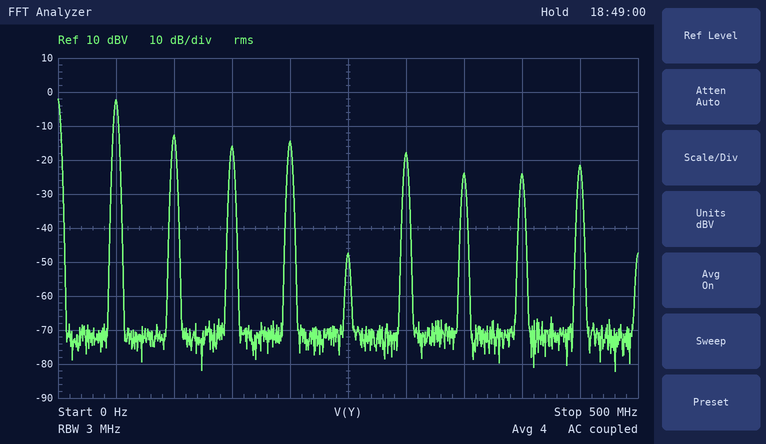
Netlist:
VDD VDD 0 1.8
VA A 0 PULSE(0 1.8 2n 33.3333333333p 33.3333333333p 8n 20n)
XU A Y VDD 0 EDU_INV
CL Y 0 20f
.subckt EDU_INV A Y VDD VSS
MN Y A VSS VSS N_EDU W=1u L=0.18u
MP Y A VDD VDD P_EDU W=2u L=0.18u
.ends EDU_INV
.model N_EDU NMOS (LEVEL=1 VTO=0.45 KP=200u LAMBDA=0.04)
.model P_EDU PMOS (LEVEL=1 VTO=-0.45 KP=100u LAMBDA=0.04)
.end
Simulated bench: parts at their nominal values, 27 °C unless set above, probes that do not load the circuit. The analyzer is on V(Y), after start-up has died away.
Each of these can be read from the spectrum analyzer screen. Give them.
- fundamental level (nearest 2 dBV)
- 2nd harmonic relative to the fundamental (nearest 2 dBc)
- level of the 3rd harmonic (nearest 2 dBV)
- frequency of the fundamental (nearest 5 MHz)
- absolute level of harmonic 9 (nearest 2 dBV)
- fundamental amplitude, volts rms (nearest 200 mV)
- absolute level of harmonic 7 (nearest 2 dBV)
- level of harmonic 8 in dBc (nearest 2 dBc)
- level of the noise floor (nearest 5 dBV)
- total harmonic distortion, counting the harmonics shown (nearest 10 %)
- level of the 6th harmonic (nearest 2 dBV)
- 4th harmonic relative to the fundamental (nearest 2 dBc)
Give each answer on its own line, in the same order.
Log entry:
-2 dBV
-10 dBc
-16 dBV
50 MHz
-22 dBV
800 mV
-24 dBV
-22 dBc
-70 dBV
50 %
-18 dBV
-12 dBc
